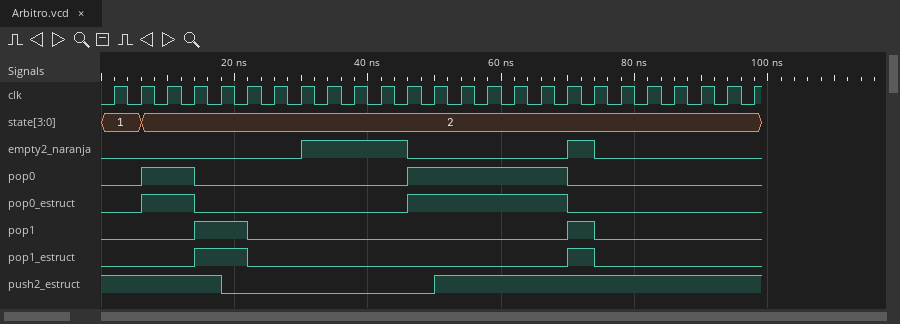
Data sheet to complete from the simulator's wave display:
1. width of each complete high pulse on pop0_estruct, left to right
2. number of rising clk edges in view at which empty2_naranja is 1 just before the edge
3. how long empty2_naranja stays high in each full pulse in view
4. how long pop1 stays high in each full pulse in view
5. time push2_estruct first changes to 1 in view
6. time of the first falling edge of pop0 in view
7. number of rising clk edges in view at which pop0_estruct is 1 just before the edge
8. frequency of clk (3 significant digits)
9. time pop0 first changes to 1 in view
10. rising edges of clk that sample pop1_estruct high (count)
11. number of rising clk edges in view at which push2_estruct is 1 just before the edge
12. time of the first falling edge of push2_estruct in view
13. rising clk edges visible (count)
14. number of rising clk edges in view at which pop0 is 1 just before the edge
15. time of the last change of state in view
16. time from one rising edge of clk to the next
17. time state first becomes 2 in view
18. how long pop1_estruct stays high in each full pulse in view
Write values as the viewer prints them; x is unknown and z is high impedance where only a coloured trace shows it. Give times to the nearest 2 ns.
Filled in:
8 ns, 24 ns
5
16 ns, 4 ns
8 ns, 4 ns
50 ns
14 ns
8
250 MHz
6 ns
3
17
18 ns
25
8
6 ns
4 ns
6 ns
8 ns, 4 ns
